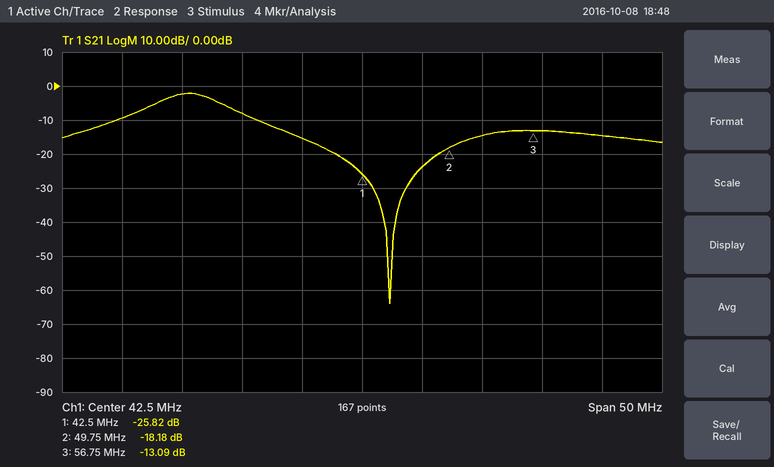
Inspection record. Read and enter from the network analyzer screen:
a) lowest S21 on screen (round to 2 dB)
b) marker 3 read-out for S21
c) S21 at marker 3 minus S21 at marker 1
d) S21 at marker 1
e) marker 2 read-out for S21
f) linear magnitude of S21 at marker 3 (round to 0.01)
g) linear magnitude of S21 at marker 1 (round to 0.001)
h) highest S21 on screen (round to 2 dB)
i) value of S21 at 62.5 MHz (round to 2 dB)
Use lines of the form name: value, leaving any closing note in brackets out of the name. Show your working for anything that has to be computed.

lowest S21 on screen: -64 dB
marker 3 read-out for S21: -13.09 dB
S21 at marker 3 minus S21 at marker 1: -13.09 − (-25.82) = 12.73 dB
S21 at marker 1: -25.82 dB
marker 2 read-out for S21: -18.18 dB
linear magnitude of S21 at marker 3: 10^(-13.09/20) ≈ 0.22
linear magnitude of S21 at marker 1: 10^(-25.82/20) ≈ 0.051
highest S21 on screen: -2 dB
value of S21 at 62.5 MHz: -14 dB
